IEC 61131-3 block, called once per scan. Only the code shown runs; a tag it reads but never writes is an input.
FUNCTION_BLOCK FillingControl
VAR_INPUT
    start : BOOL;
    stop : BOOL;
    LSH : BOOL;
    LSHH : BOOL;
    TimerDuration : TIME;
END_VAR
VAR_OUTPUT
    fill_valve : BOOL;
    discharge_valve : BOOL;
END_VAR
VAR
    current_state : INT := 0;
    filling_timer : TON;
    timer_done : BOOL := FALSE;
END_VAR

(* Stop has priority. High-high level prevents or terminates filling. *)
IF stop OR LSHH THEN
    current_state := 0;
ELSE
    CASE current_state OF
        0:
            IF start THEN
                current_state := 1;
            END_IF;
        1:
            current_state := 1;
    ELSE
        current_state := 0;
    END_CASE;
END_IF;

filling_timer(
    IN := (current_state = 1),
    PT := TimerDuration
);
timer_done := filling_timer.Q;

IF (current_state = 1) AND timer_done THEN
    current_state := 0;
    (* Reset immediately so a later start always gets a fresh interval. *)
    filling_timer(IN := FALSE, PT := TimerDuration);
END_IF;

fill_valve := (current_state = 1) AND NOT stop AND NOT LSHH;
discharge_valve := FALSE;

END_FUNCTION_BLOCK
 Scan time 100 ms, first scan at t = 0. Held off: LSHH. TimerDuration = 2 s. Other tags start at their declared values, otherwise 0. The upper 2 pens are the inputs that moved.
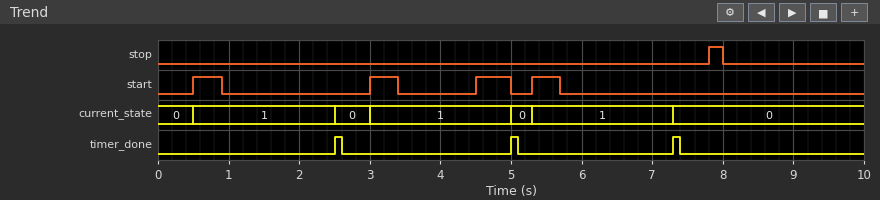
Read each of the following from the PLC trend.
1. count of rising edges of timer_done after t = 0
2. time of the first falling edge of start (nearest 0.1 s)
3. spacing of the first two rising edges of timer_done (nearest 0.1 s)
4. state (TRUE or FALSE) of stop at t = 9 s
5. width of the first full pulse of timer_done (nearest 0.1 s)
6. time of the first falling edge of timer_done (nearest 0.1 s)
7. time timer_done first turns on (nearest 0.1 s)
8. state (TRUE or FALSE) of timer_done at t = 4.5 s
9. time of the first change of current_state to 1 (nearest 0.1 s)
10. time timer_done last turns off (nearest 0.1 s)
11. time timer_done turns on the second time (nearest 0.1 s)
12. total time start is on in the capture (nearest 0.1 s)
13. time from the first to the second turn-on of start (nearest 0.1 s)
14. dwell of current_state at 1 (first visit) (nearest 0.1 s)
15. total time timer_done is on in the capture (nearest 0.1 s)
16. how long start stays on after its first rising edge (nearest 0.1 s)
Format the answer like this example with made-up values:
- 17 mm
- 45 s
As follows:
- 3
- 0.9 s
- 2.5 s
- FALSE
- 0.1 s
- 2.6 s
- 2.5 s
- FALSE
- 0.5 s
- 7.4 s
- 5.0 s
- 1.7 s
- 2.5 s
- 2.0 s
- 0.3 s
- 0.4 s
